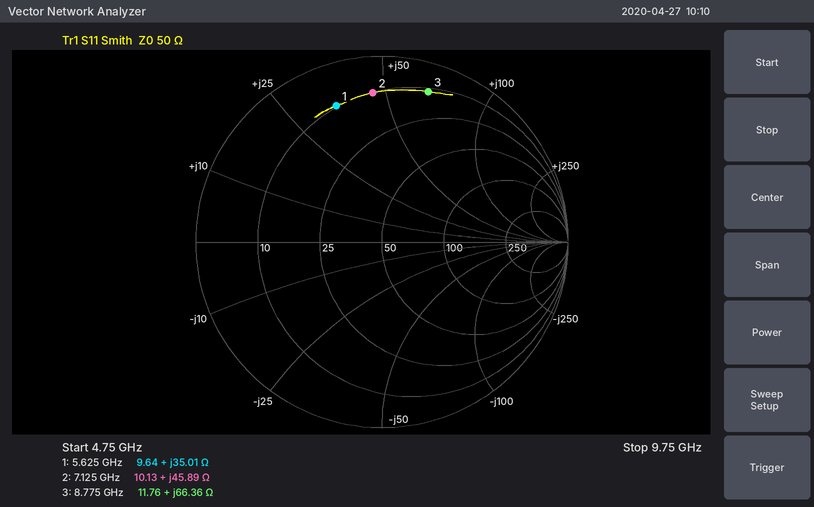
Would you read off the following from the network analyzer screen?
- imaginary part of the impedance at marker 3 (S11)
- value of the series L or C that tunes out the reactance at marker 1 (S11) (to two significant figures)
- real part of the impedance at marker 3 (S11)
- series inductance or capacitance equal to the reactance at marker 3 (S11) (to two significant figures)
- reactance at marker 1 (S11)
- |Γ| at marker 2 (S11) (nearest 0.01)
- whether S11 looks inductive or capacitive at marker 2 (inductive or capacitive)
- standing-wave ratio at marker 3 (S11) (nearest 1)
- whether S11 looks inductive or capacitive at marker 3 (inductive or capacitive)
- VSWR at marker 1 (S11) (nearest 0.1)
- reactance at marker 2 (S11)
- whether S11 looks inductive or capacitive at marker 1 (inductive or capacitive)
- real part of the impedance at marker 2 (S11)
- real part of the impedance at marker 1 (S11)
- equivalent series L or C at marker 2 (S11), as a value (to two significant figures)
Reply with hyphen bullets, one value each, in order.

- +66.36 Ω
- 810 fF
- 11.76 Ω
- 1.2 nH
- +35.01 Ω
- 0.80
- inductive
- 12
- inductive
- 7.8
- +45.89 Ω
- inductive
- 10.13 Ω
- 9.64 Ω
- 1.0 nH
